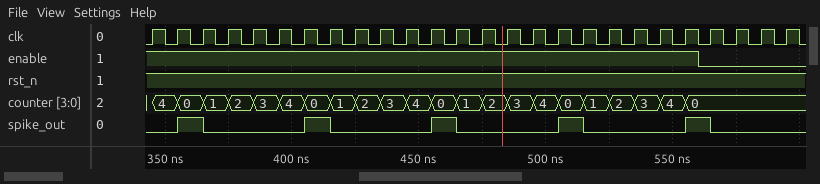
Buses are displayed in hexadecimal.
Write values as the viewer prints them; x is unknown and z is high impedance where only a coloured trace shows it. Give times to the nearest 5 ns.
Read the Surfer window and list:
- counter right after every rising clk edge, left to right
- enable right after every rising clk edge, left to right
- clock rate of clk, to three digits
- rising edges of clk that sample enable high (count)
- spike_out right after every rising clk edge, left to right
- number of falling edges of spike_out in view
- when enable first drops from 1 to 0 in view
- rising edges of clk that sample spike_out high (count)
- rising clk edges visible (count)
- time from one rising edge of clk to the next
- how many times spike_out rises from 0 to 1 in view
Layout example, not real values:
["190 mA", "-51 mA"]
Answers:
["4, 0, 1, 2, 3, 4, 0, 1, 2, 3, 4, 0, 1, 2, 3, 4, 0, 1, 2, 3, 4, 0, 0, 0, 0, 0", "1 1 1 1 1 1 1 1 1 1 1 1 1 1 1 1 1 1 1 1 1 1 0 0 0 0", "100 MHz", "22", "0 1 0 0 0 0 1 0 0 0 0 1 0 0 0 0 1 0 0 0 0 1 0 0 0 0", "5", "560 ns", "5", "26", "10 ns", "5"]
